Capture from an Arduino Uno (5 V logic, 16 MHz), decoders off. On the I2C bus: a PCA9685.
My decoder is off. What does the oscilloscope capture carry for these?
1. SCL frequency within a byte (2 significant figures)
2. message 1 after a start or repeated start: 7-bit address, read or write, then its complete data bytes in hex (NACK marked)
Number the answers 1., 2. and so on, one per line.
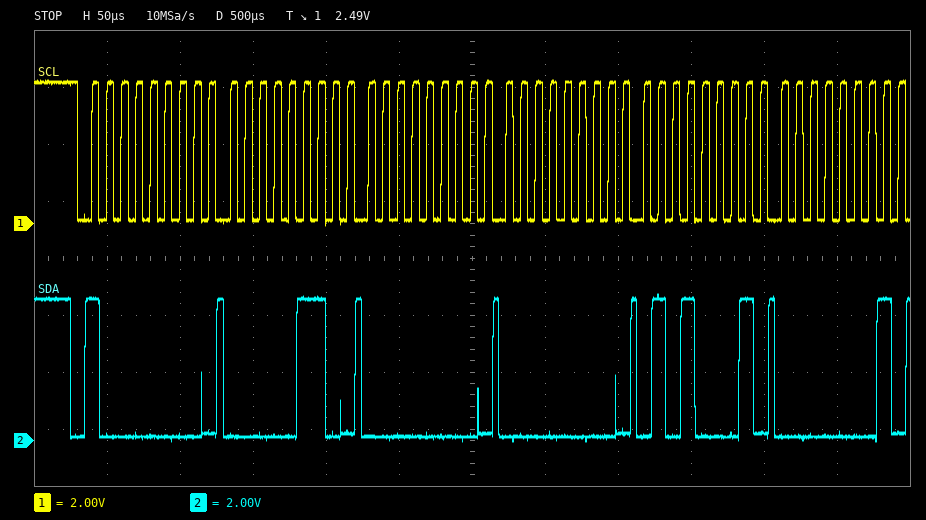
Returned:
1. 100 kHz
2. 0x40 write: 06 00 00 51 01
